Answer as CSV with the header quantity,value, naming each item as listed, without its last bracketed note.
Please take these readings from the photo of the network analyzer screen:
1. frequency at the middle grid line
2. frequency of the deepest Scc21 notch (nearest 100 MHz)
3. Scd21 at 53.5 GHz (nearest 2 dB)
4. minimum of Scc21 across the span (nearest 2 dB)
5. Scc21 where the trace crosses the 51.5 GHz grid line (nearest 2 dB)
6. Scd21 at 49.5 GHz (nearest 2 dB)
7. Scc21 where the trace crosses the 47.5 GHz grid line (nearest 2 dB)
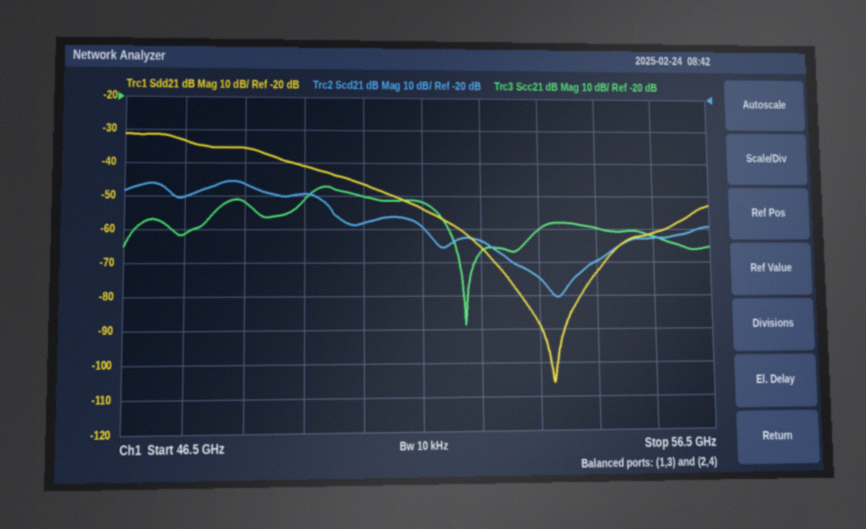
quantity,value
frequency at the middle grid line,51.5 GHz
frequency of the deepest Scc21 notch,52.2 GHz
Scd21 at 53.5 GHz,-74 dB
minimum of Scc21 across the span,-88 dB
Scc21 where the trace crosses the 51.5 GHz grid line,-52 dB
Scd21 at 49.5 GHz,-50 dB
Scc21 where the trace crosses the 47.5 GHz grid line,-62 dB
